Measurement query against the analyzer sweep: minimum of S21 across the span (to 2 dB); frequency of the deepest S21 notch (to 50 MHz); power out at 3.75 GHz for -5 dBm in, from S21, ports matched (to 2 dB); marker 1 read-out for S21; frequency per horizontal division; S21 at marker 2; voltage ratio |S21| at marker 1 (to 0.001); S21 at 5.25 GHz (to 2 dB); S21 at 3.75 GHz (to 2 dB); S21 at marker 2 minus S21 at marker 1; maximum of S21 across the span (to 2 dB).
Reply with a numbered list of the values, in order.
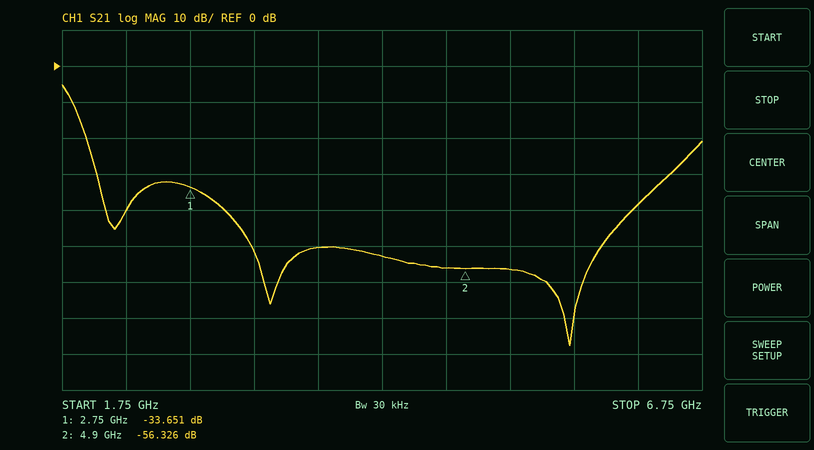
1. -78 dB
2. 5.70 GHz
3. -56 dBm
4. -33.651 dB
5. 500 MHz
6. -56.326 dB
7. 0.021
8. -56 dB
9. -50 dB
10. -22.675 dB
11. -6 dB
